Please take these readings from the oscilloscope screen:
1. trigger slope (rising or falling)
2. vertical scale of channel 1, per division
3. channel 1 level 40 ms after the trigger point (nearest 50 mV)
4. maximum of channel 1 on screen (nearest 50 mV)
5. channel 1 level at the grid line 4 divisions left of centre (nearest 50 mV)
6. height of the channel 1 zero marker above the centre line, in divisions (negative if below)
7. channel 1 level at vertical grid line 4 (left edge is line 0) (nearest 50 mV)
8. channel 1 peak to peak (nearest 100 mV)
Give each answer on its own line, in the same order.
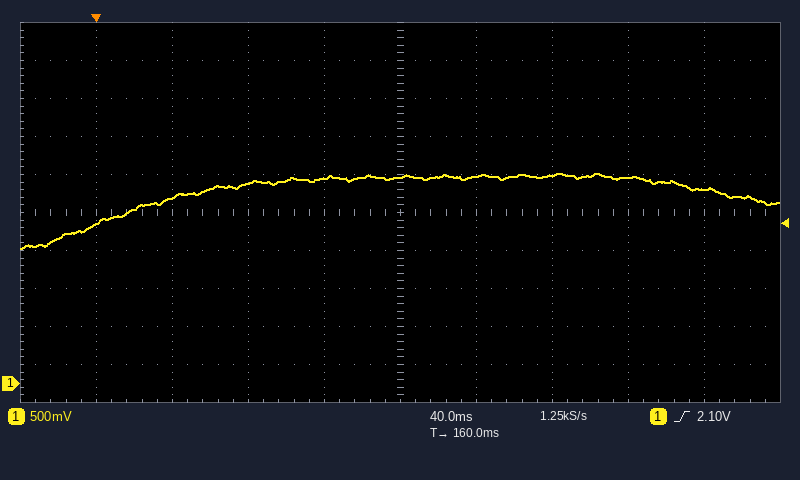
rising
500 mV
2.45 V
2.75 V
2.10 V
-4.5 div
2.70 V
1.00 V
